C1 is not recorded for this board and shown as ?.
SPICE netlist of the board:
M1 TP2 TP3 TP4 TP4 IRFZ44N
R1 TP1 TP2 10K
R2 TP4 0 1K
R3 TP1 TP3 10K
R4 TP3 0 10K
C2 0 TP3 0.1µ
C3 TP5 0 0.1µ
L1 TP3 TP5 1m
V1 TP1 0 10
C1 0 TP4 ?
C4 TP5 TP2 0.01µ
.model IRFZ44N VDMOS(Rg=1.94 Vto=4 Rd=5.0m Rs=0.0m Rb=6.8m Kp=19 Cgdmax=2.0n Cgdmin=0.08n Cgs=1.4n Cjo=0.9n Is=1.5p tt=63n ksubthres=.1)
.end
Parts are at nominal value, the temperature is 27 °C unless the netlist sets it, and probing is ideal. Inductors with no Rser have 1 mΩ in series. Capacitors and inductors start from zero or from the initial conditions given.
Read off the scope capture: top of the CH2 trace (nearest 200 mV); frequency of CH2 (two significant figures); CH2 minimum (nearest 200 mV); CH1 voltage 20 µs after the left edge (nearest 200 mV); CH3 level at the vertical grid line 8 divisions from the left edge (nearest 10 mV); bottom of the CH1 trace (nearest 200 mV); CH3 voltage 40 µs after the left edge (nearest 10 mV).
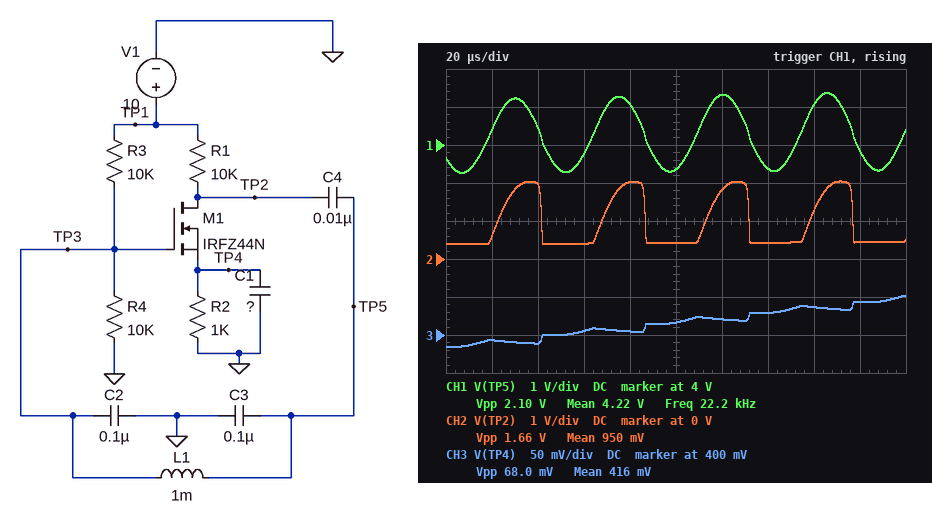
2.0 V
22 kHz
400 mV
4.4 V
440 mV
3.2 V
390 mV
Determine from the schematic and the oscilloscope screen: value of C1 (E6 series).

1.5 µF
